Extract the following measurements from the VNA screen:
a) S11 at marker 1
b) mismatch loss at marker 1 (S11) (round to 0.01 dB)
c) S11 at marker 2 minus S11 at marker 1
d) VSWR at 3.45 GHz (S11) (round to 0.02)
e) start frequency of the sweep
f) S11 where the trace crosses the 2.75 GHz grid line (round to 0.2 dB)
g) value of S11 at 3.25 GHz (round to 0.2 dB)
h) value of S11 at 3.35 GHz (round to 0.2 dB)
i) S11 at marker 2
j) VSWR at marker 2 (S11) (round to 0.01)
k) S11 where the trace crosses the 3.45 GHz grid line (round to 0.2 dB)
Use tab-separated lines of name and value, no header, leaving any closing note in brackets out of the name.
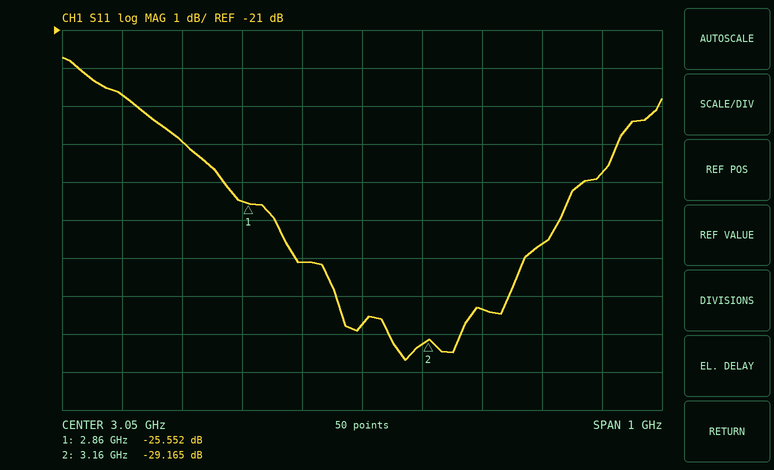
S11 at marker 1	-25.552 dB
mismatch loss at marker 1 (S11)	0.01 dB
S11 at marker 2 minus S11 at marker 1	-3.613 dB
VSWR at 3.45 GHz (S11)	1.12
start frequency of the sweep	2.55 GHz
S11 where the trace crosses the 2.75 GHz grid line	-24.0 dB
value of S11 at 3.25 GHz	-28.4 dB
value of S11 at 3.35 GHz	-26.6 dB
S11 at marker 2	-29.165 dB
VSWR at marker 2 (S11)	1.07
S11 where the trace crosses the 3.45 GHz grid line	-24.8 dB
